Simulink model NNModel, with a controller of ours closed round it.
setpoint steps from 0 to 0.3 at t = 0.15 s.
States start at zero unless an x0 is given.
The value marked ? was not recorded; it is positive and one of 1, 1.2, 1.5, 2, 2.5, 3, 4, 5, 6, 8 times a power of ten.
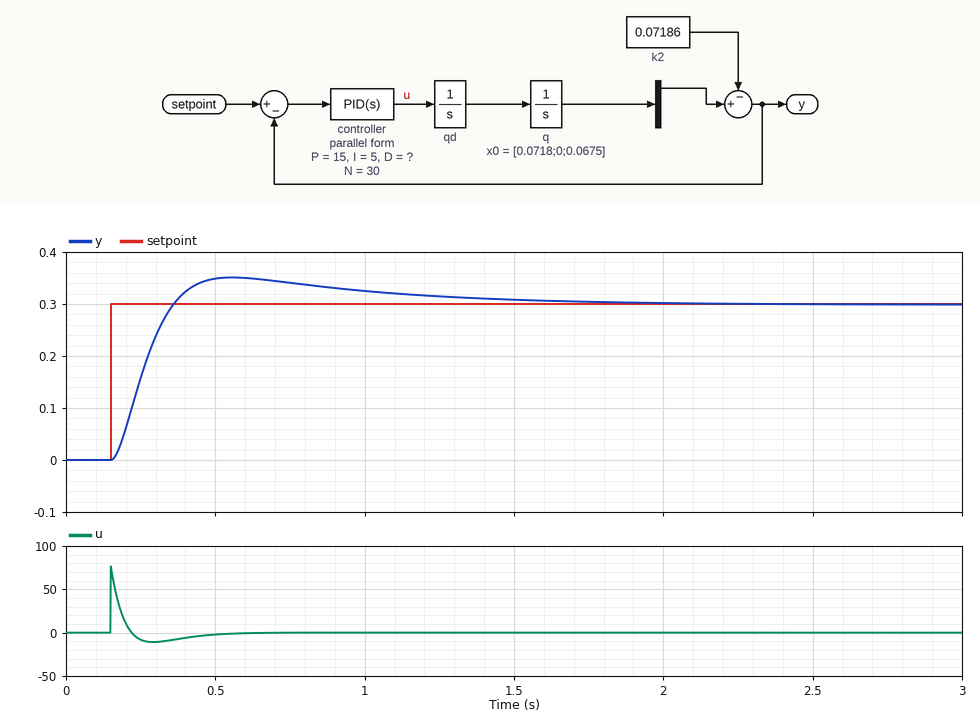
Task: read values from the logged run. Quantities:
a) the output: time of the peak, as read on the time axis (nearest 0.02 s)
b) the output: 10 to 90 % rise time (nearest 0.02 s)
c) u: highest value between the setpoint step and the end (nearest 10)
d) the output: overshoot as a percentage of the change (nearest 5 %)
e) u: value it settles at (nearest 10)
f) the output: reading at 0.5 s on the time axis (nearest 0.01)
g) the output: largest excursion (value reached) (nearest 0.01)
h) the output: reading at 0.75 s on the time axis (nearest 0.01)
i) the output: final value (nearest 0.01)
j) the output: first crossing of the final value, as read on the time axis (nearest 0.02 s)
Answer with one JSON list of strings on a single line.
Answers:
["0.56 s", "0.14 s", "80", "15 %", "0", "0.35", "0.35", "0.34", "0.30", "0.36 s"]
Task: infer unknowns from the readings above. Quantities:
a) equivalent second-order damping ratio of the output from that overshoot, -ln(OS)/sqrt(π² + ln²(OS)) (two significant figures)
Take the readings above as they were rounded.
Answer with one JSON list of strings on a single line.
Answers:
["0.52"]
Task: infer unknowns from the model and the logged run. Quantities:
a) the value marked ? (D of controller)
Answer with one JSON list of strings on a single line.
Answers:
["8"]
